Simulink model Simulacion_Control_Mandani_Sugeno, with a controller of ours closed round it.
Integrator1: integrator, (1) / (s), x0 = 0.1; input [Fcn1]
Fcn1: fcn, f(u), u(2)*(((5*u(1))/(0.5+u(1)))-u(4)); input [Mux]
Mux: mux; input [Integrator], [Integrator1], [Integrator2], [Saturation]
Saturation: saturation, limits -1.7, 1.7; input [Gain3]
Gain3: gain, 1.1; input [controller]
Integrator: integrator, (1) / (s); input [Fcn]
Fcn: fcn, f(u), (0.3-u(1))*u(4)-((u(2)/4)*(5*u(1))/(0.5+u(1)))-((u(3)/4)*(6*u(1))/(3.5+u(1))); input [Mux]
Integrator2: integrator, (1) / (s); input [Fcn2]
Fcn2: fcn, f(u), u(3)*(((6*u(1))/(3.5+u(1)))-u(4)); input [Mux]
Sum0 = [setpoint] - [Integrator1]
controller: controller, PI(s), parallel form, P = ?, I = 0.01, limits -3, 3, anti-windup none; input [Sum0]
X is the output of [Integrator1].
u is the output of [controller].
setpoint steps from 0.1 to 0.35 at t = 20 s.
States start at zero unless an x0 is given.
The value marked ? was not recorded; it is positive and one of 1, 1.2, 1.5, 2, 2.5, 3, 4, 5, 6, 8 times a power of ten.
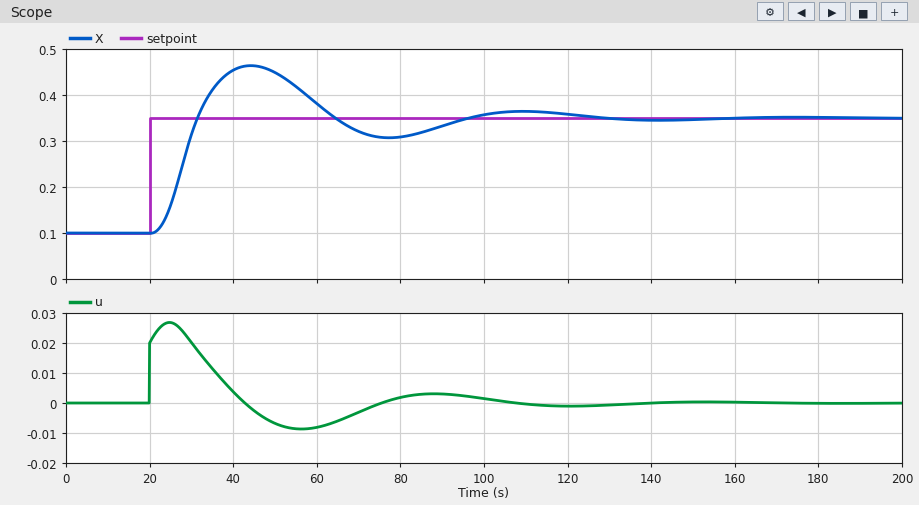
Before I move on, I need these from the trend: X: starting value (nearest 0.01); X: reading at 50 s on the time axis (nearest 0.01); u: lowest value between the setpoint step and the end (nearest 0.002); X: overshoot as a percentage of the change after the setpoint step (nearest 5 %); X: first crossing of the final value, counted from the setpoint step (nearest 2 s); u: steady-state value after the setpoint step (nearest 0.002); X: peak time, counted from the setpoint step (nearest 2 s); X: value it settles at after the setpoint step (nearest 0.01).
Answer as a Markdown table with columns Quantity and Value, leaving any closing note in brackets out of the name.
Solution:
| Quantity | Value |
|---|---|
| X: starting value | 0.10 |
| X: reading at 50 s on the time axis | 0.45 |
| u: lowest value between the setpoint step and the end | -0.008 |
| X: overshoot as a percentage of the change after the setpoint step | 45 % |
| X: first crossing of the final value, counted from the setpoint step | 12 s |
| u: steady-state value after the setpoint step | 0.000 |
| X: peak time, counted from the setpoint step | 24 s |
| X: value it settles at after the setpoint step | 0.35 |
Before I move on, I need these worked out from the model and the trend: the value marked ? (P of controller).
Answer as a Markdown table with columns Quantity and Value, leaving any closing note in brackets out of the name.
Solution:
| Quantity | Value |
|---|---|
| the value marked ? | 0.08 |
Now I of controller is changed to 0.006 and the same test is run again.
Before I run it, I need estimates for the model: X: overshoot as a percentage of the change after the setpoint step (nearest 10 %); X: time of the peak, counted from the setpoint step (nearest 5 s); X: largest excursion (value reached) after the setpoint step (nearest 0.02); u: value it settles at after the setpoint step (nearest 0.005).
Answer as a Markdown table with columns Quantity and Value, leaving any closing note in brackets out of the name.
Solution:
| Quantity | Value |
|---|---|
| X: overshoot as a percentage of the change after the setpoint step | 30 % |
| X: time of the peak, counted from the setpoint step | 30 s |
| X: largest excursion (value reached) after the setpoint step | 0.44 |
| u: value it settles at after the setpoint step | 0.000 |
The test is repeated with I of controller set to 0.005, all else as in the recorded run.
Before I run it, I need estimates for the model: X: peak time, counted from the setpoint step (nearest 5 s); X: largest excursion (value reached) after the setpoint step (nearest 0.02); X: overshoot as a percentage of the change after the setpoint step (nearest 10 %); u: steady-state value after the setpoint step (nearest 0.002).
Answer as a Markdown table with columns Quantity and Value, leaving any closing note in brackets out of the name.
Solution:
| Quantity | Value |
|---|---|
| X: peak time, counted from the setpoint step | 30 s |
| X: largest excursion (value reached) after the setpoint step | 0.42 |
| X: overshoot as a percentage of the change after the setpoint step | 30 % |
| u: steady-state value after the setpoint step | 0.000 |
